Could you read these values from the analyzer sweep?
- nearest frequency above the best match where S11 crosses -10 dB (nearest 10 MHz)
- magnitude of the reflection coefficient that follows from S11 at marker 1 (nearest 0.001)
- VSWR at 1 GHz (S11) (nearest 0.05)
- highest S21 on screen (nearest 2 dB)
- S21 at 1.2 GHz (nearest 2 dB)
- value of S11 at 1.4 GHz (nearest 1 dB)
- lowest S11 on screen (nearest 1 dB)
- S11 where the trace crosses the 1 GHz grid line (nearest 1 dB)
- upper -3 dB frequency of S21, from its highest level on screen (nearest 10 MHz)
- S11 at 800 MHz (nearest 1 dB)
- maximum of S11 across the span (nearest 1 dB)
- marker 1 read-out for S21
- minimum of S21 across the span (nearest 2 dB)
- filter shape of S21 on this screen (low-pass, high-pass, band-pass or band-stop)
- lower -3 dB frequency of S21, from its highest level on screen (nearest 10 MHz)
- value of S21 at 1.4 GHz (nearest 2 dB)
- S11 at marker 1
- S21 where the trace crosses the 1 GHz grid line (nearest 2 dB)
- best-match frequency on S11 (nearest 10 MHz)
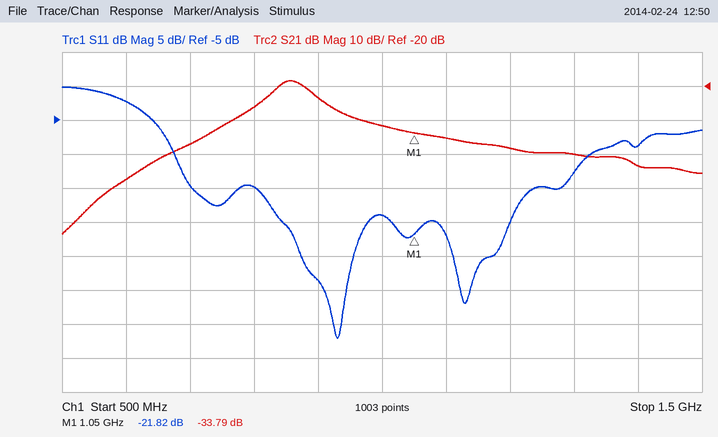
1.33 GHz
0.081
1.25
-18 dB
-38 dB
-9 dB
-37 dB
-19 dB
890 MHz
-15 dB
0 dB
-33.79 dB
-64 dB
band-pass
830 MHz
-44 dB
-21.82 dB
-32 dB
930 MHz
